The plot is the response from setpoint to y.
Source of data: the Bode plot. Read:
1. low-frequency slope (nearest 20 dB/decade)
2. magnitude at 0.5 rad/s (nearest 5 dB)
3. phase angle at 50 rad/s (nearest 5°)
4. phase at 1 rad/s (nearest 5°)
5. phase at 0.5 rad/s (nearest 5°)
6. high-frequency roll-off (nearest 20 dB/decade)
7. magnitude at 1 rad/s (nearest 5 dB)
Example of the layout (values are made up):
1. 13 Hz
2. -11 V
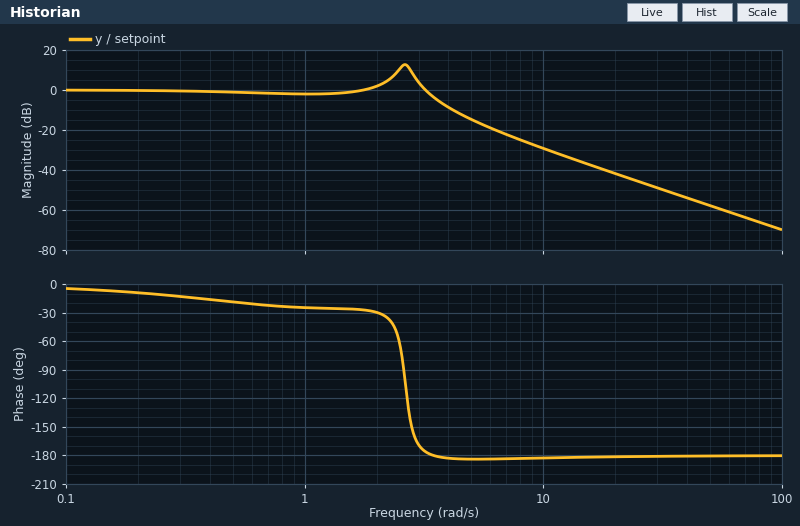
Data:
1. 0 dB/decade
2. 0 dB
3. -180°
4. -25°
5. -20°
6. -40 dB/decade
7. 0 dB
